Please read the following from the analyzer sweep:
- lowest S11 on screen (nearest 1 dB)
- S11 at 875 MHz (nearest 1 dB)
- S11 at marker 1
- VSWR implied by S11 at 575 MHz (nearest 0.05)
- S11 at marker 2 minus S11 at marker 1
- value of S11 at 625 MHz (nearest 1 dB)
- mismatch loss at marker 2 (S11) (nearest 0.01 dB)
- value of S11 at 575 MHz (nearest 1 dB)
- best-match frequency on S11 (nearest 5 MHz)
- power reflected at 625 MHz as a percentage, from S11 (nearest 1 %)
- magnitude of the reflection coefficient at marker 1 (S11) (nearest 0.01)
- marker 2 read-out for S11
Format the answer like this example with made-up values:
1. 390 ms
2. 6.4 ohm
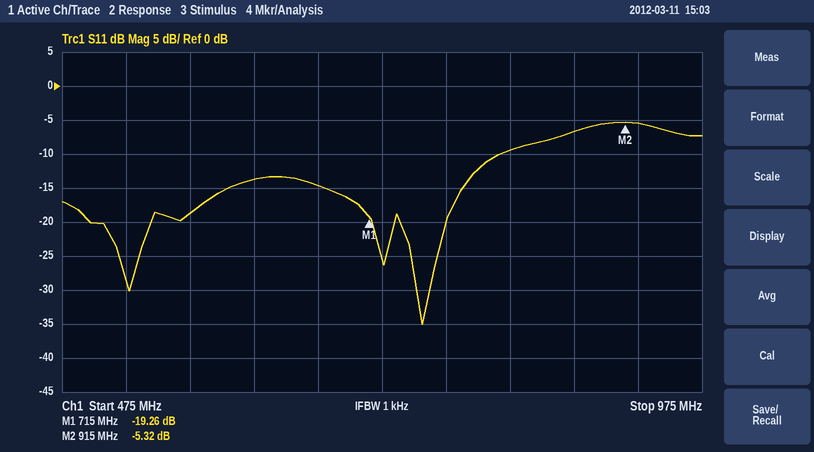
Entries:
1. -35 dB
2. -7 dB
3. -19.26 dB
4. 1.25
5. 13.94 dB
6. -14 dB
7. 1.51 dB
8. -19 dB
9. 755 MHz
10. 4 %
11. 0.11
12. -5.32 dB
